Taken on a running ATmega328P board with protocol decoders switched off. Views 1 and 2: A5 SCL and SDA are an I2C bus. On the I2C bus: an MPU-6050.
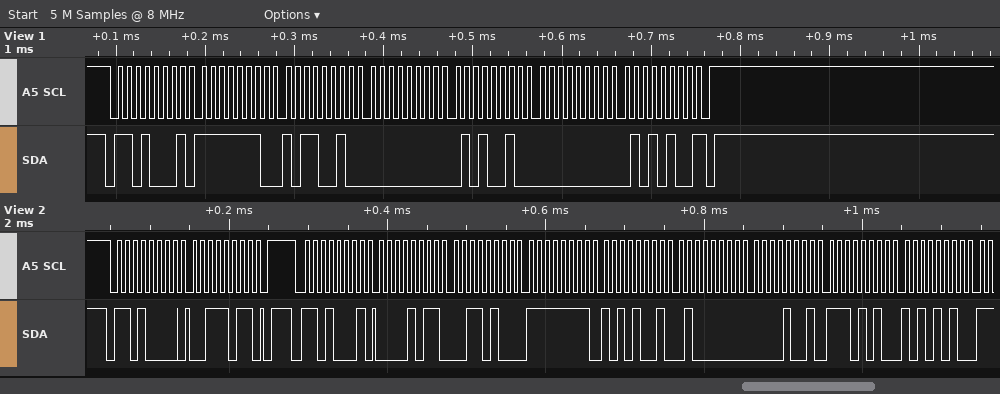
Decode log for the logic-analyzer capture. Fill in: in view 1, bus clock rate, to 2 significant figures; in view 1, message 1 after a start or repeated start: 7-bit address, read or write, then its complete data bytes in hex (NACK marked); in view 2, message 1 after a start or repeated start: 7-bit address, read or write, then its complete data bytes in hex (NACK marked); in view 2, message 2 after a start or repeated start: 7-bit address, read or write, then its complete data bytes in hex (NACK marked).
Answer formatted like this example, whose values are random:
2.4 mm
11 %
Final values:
100 kHz
0x68 read: FE B2 00 52 00 54 NACK
0x68 write: 3B
0x68 read: 0B 34 FF A9 40 09 EA AA
